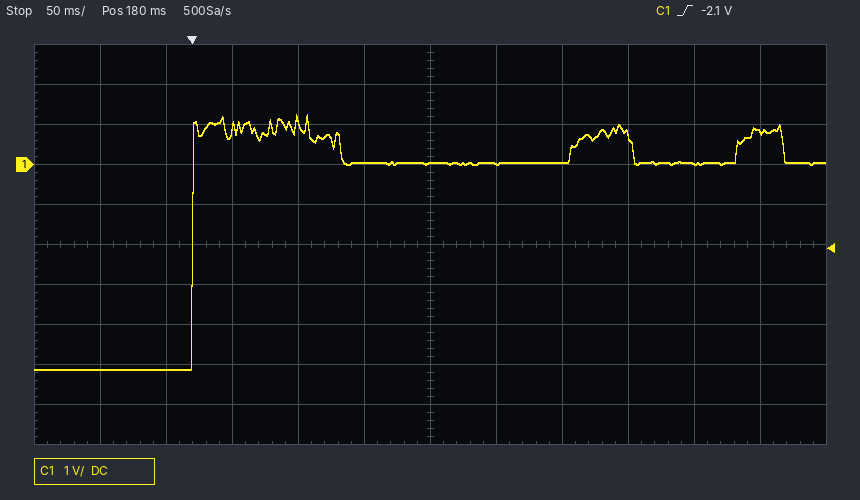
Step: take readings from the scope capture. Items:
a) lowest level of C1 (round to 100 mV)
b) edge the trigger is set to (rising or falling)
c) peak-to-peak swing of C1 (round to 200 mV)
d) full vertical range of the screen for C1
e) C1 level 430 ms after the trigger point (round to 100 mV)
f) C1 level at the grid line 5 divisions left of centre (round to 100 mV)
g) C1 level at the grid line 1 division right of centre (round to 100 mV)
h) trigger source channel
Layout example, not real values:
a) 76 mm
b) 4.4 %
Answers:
a) -5.1 V
b) rising
c) 6.4 V
d) 10 V
e) 800 mV
f) -5.1 V
g) 0.0 V
h) C1
